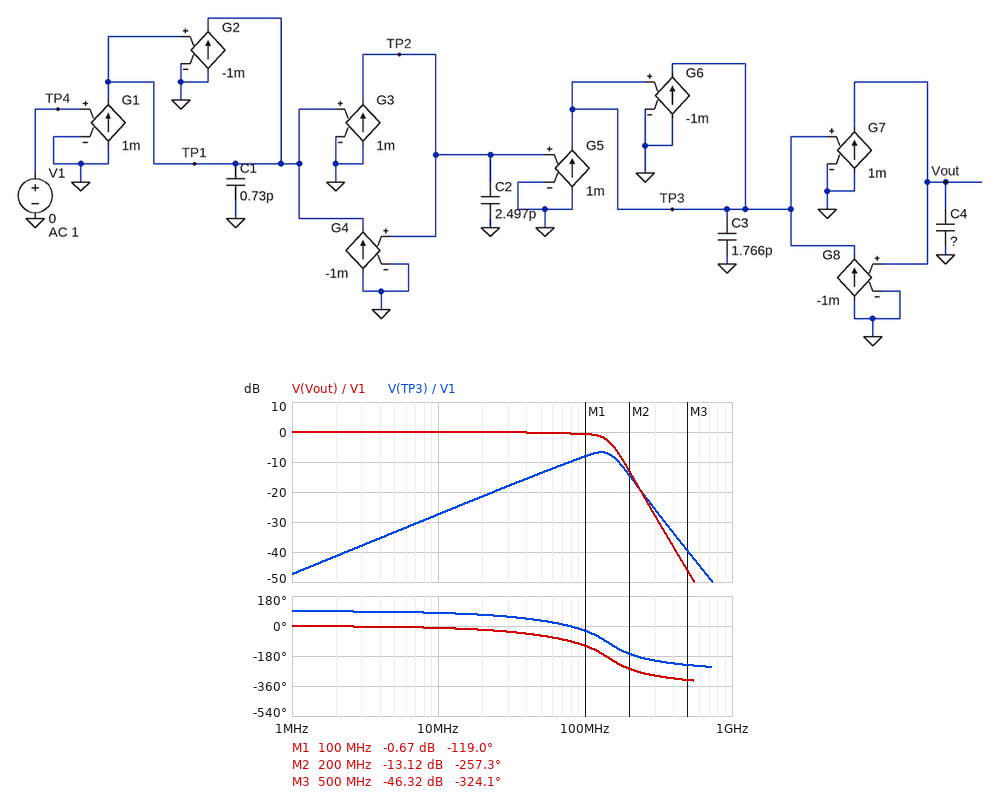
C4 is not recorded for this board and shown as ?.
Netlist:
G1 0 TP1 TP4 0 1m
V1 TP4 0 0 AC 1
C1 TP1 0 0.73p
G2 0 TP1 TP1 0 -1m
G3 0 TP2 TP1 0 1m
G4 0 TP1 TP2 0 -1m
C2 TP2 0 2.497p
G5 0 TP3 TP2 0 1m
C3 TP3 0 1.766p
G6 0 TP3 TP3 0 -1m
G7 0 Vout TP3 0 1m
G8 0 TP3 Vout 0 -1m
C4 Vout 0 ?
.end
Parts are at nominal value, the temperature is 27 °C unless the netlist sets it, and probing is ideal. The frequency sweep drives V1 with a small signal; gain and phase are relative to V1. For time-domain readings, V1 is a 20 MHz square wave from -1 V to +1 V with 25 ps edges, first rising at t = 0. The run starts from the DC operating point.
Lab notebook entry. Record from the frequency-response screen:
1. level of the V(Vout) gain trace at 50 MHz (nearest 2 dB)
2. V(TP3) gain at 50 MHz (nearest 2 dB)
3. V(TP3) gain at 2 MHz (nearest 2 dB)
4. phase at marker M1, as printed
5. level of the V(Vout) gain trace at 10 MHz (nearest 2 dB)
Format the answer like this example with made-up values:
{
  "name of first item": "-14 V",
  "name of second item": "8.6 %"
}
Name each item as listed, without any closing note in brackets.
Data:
{
  "level of the V(Vout) gain trace at 50 MHz": "0 dB",
  "V(TP3) gain at 50 MHz": "-14 dB",
  "V(TP3) gain at 2 MHz": "-42 dB",
  "phase at marker M1, as printed": "-119.0 deg",
  "level of the V(Vout) gain trace at 10 MHz": "0 dB"
}
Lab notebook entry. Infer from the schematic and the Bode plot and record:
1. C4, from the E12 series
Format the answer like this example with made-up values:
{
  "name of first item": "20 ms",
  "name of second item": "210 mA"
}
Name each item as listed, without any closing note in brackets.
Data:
{
  "C4, from the E12 series": "680 fF"
}
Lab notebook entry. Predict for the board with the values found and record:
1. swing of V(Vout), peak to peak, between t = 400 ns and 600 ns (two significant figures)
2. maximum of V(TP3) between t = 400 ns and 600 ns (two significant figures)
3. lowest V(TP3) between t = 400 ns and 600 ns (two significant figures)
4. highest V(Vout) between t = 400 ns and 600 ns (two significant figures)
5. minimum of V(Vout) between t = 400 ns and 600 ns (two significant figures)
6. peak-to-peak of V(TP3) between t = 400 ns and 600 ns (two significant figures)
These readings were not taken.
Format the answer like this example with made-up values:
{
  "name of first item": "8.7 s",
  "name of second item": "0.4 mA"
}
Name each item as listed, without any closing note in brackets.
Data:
{
  "swing of V(Vout), peak to peak, between t = 400 ns and 600 ns": "2.4 V",
  "maximum of V(TP3) between t = 400 ns and 600 ns": "450 mV",
  "lowest V(TP3) between t = 400 ns and 600 ns": "-450 mV",
  "highest V(Vout) between t = 400 ns and 600 ns": "1.2 V",
  "minimum of V(Vout) between t = 400 ns and 600 ns": "-1.2 V",
  "peak-to-peak of V(TP3) between t = 400 ns and 600 ns": "900 mV"
}
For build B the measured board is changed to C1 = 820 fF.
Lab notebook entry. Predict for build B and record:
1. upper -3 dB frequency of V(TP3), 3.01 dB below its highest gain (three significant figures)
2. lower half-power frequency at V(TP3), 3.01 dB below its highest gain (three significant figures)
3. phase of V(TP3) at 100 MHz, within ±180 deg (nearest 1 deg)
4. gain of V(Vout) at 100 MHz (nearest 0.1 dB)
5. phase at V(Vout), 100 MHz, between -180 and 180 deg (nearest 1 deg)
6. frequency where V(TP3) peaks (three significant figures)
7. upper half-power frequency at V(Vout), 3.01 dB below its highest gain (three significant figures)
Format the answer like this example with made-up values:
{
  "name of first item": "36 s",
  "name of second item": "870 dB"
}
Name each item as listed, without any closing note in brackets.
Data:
{
  "upper -3 dB frequency of V(TP3), 3.01 dB below its highest gain": "165 MHz",
  "lower half-power frequency at V(TP3), 3.01 dB below its highest gain": "78.5 MHz",
  "phase of V(TP3) at 100 MHz, within ±180 deg": "-32 deg",
  "gain of V(Vout) at 100 MHz": "-0.6 dB",
  "phase at V(Vout), 100 MHz, between -180 and 180 deg": "-122 deg",
  "frequency where V(TP3) peaks": "127 MHz",
  "upper half-power frequency at V(Vout), 3.01 dB below its highest gain": "142 MHz"
}
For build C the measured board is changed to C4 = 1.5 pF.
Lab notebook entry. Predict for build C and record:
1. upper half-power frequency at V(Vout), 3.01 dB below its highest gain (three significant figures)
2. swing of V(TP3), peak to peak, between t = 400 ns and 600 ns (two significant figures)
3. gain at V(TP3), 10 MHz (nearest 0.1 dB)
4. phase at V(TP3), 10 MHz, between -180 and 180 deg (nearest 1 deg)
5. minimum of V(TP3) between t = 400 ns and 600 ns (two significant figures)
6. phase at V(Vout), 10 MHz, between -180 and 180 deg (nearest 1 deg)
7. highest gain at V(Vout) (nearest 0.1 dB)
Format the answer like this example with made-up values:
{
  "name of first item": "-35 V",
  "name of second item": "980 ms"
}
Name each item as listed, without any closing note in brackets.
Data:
{
  "upper half-power frequency at V(Vout), 3.01 dB below its highest gain": "96.2 MHz",
  "swing of V(TP3), peak to peak, between t = 400 ns and 600 ns": "1.4 V",
  "gain at V(TP3), 10 MHz": "-20.5 dB",
  "phase at V(TP3), 10 MHz, between -180 and 180 deg": "76 deg",
  "minimum of V(TP3) between t = 400 ns and 600 ns": "-720 mV",
  "phase at V(Vout), 10 MHz, between -180 and 180 deg": "-14 deg",
  "highest gain at V(Vout)": "0.1 dB"
}
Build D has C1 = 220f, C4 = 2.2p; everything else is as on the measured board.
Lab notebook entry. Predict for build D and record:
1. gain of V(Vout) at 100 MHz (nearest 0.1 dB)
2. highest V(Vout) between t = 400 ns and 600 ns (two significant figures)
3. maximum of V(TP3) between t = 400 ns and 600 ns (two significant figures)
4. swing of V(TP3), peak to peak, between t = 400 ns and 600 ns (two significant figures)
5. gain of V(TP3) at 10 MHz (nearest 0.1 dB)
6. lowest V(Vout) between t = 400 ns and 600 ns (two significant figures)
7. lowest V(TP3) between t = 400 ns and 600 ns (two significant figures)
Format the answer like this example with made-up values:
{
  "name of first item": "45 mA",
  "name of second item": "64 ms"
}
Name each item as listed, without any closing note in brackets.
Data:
{
  "gain of V(Vout) at 100 MHz": "-8.3 dB",
  "highest V(Vout) between t = 400 ns and 600 ns": "1.1 V",
  "maximum of V(TP3) between t = 400 ns and 600 ns": "810 mV",
  "swing of V(TP3), peak to peak, between t = 400 ns and 600 ns": "1.6 V",
  "gain of V(TP3) at 10 MHz": "-17.2 dB",
  "lowest V(Vout) between t = 400 ns and 600 ns": "-1.1 V",
  "lowest V(TP3) between t = 400 ns and 600 ns": "-810 mV"
}
